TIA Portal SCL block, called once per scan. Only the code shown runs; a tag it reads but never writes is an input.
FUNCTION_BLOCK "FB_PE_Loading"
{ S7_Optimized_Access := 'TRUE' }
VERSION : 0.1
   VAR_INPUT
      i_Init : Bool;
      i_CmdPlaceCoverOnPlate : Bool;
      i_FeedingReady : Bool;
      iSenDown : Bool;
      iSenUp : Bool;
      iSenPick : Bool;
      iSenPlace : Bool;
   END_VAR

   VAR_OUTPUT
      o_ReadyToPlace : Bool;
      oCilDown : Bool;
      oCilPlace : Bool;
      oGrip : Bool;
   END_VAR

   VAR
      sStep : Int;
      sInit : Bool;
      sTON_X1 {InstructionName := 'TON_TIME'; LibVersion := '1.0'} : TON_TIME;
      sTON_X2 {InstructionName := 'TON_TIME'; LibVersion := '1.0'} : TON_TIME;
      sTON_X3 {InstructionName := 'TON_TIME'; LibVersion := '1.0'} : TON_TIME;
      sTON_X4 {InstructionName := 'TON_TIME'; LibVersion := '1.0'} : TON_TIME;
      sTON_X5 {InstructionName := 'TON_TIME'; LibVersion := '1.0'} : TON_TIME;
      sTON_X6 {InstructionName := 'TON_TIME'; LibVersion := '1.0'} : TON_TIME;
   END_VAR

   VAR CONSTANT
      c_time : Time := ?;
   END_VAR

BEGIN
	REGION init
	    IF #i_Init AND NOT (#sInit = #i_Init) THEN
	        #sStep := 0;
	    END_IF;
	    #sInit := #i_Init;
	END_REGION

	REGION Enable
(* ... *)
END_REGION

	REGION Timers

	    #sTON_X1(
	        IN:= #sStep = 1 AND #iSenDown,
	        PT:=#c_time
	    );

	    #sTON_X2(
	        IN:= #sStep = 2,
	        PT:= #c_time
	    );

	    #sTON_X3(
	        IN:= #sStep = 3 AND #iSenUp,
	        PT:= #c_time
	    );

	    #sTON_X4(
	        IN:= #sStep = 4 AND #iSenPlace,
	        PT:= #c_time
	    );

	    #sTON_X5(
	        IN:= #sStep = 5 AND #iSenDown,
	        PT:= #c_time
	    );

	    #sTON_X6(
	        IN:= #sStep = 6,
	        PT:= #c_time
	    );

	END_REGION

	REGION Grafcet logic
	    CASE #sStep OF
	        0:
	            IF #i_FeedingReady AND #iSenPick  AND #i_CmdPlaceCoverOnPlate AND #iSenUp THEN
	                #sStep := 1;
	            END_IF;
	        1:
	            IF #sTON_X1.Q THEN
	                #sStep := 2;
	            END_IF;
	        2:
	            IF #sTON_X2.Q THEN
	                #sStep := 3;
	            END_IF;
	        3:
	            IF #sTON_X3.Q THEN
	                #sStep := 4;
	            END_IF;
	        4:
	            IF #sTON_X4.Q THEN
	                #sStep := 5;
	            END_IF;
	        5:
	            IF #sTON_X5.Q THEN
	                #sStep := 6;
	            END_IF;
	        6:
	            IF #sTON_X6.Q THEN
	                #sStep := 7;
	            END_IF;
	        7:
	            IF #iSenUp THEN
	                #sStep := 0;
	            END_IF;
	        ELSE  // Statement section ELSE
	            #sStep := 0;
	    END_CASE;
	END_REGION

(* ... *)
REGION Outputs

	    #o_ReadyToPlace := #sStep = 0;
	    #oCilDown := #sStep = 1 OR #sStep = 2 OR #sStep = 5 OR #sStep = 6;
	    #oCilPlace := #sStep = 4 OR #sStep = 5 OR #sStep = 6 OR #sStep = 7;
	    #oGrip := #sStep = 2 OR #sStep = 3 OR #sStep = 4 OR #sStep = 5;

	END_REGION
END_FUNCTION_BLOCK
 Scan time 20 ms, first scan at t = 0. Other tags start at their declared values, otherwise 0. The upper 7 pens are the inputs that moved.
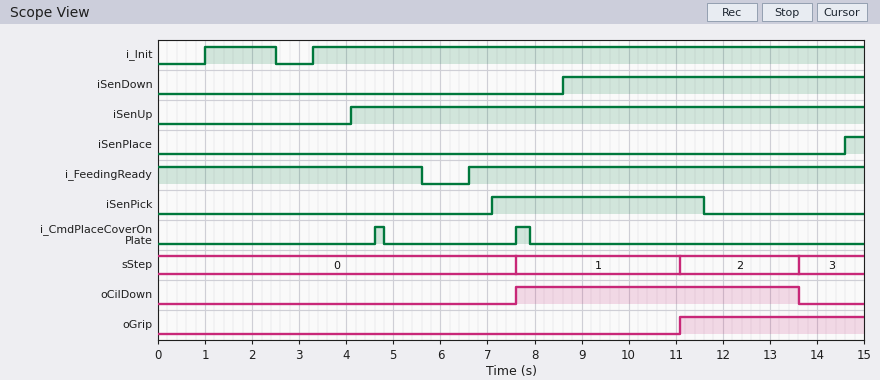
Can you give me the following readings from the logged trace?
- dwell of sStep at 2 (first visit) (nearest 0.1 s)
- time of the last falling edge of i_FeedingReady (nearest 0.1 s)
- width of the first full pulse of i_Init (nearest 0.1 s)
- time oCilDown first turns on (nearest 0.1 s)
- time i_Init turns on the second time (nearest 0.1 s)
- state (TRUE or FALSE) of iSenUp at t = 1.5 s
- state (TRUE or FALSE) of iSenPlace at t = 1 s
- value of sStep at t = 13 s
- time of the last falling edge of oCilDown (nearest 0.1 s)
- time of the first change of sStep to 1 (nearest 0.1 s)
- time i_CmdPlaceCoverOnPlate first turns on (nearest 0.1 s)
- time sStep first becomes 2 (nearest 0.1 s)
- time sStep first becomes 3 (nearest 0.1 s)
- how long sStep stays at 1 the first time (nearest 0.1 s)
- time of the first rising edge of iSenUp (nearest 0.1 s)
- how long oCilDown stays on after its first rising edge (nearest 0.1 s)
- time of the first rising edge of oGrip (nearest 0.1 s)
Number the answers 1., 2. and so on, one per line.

1. 2.5 s
2. 5.6 s
3. 1.5 s
4. 7.6 s
5. 3.3 s
6. FALSE
7. FALSE
8. 2
9. 13.6 s
10. 7.6 s
11. 4.6 s
12. 11.1 s
13. 13.6 s
14. 3.5 s
15. 4.1 s
16. 6.0 s
17. 11.1 s
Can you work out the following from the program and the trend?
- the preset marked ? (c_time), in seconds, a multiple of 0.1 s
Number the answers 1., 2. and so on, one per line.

1. 2.5 s
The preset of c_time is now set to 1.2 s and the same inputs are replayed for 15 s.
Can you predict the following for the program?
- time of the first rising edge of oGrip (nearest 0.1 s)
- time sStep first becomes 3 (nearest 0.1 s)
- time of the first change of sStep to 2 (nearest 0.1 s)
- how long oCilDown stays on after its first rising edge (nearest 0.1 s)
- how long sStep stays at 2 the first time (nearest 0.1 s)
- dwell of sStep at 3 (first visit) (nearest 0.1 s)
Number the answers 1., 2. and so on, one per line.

1. 9.8 s
2. 11.0 s
3. 9.8 s
4. 3.4 s
5. 1.2 s
6. 1.2 s
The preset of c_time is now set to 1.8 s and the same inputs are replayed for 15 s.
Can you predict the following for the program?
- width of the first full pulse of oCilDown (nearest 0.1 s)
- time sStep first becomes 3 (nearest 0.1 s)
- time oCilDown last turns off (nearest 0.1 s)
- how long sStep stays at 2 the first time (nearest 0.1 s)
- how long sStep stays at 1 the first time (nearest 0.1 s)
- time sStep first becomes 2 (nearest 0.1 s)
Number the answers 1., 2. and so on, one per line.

1. 4.6 s
2. 12.2 s
3. 12.2 s
4. 1.8 s
5. 2.8 s
6. 10.4 s
